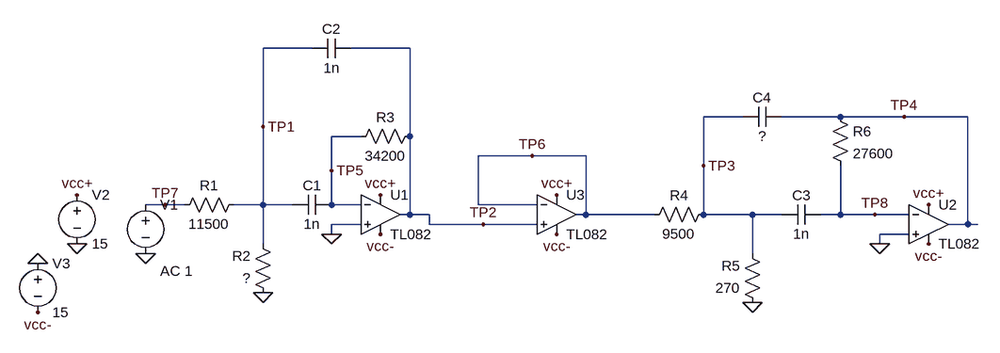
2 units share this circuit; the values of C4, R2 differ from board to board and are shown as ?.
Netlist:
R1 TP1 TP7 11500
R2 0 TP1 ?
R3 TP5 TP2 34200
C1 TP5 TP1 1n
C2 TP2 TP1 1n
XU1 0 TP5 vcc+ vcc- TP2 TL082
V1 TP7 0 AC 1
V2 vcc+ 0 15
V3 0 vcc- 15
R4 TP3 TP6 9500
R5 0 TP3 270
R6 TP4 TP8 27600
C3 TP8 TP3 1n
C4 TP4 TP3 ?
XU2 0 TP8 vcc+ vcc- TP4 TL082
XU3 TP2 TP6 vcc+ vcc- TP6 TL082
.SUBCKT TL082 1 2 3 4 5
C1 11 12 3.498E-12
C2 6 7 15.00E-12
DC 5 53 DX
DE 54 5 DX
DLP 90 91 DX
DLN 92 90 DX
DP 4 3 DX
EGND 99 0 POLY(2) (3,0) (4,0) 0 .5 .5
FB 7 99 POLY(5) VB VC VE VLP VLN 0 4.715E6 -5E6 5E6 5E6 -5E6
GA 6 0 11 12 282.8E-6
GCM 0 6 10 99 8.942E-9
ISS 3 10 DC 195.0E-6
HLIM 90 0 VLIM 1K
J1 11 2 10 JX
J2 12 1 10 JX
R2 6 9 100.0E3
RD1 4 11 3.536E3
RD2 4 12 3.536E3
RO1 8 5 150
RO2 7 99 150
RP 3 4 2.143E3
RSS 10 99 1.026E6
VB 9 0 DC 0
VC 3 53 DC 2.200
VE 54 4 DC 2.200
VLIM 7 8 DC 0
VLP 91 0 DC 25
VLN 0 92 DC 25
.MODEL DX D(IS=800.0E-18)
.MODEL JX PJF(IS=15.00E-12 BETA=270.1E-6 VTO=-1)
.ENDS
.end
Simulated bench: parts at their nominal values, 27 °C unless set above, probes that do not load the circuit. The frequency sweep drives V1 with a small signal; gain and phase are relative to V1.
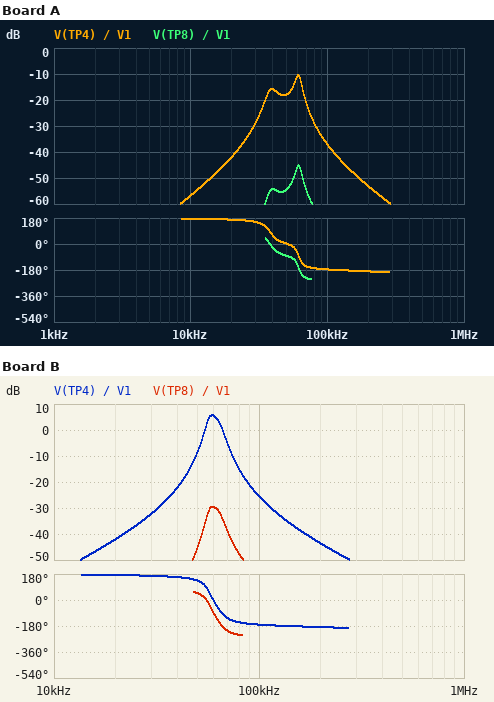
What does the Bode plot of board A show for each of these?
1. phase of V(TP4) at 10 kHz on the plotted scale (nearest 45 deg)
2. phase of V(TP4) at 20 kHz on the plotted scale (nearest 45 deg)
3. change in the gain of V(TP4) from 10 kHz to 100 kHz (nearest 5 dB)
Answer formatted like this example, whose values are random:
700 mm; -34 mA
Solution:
180 deg; 180 deg; 20 dB
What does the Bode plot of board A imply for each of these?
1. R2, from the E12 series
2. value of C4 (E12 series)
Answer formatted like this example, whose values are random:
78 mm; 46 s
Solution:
150 Ω; 2.2 nF
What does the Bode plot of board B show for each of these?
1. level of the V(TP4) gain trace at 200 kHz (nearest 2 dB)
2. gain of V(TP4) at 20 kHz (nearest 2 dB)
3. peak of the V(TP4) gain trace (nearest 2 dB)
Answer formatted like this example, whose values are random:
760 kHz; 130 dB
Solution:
-44 dB; -42 dB; 6 dB
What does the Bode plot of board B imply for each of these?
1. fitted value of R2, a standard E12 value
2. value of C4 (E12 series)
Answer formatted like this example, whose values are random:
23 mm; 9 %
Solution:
180 Ω; 680 pF
